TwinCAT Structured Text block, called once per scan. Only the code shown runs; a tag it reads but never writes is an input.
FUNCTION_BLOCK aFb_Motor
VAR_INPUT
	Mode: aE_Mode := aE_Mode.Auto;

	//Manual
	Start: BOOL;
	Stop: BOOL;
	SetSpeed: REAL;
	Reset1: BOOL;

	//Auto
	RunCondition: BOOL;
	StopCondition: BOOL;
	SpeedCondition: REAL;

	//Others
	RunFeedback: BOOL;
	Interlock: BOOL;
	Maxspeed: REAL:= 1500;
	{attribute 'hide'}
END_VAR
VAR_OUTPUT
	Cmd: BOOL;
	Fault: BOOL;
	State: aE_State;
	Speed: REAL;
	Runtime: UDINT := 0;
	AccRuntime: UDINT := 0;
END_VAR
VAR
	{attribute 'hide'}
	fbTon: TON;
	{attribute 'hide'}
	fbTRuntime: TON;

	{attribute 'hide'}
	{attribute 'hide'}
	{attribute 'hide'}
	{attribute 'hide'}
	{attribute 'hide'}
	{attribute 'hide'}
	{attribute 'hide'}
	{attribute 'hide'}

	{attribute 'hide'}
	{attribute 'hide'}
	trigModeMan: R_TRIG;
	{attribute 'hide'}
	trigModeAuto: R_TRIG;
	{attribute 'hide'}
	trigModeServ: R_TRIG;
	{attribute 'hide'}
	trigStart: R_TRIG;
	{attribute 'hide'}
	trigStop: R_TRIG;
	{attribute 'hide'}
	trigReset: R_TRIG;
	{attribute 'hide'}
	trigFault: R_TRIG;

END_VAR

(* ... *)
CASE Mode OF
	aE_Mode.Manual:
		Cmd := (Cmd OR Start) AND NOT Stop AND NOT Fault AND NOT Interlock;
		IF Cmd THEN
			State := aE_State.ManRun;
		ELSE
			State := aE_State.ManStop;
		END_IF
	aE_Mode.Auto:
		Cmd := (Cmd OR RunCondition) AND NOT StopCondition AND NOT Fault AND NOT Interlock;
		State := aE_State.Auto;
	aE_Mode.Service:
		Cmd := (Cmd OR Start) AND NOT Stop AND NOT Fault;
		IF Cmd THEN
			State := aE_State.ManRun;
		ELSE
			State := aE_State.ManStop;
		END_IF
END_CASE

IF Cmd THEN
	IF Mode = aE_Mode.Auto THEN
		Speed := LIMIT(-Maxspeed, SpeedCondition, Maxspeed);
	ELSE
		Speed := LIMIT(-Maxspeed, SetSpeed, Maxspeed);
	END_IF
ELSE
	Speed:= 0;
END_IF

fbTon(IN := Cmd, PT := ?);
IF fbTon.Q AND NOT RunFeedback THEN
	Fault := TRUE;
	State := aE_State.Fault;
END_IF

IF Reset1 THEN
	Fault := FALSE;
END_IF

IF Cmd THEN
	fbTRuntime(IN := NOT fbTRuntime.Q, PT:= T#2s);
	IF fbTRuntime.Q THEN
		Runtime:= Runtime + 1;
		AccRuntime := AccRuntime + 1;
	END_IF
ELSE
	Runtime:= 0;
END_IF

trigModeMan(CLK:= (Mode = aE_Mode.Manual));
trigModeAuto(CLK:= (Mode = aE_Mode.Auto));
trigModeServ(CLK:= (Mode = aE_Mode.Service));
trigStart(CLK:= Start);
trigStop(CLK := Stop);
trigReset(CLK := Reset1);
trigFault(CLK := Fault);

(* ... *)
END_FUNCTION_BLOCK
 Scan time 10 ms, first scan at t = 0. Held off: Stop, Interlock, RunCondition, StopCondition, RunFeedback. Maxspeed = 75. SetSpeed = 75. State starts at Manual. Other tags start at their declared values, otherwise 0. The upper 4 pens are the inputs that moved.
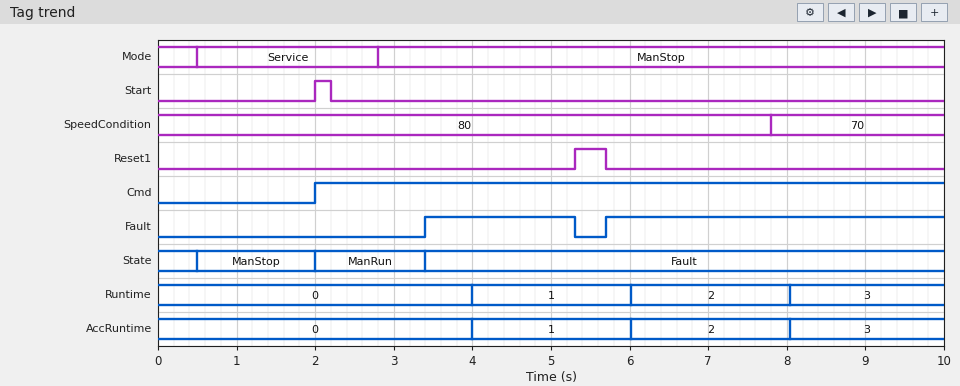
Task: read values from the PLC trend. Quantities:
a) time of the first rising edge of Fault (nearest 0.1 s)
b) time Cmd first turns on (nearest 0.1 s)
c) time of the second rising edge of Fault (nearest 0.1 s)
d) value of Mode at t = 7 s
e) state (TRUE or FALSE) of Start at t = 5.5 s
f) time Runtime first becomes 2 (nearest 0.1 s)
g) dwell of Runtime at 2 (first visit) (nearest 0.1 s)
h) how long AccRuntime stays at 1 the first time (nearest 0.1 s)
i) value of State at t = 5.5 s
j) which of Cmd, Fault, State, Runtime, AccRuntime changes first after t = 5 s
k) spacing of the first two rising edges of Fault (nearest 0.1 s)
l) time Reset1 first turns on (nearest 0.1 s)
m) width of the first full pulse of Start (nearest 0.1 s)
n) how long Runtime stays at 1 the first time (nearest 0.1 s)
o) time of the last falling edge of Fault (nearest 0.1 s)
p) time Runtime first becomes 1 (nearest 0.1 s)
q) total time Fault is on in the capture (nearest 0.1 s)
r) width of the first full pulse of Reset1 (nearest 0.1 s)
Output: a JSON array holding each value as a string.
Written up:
["3.4 s", "2.0 s", "5.7 s", "ManStop", "FALSE", "6.0 s", "2.0 s", "2.0 s", "Fault", "Fault", "2.3 s", "5.3 s", "0.2 s", "2.0 s", "5.3 s", "4.0 s", "6.2 s", "0.4 s"]
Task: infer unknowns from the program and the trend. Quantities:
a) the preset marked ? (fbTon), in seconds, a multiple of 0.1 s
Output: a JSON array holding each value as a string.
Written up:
["1.4 s"]
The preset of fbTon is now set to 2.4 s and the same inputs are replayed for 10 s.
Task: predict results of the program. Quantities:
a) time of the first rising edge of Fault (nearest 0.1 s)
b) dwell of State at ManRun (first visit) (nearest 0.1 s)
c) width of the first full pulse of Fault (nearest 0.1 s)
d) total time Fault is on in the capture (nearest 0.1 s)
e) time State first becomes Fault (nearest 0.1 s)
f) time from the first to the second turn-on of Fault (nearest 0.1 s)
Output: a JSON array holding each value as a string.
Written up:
["4.4 s", "2.4 s", "0.9 s", "5.2 s", "4.4 s", "1.3 s"]
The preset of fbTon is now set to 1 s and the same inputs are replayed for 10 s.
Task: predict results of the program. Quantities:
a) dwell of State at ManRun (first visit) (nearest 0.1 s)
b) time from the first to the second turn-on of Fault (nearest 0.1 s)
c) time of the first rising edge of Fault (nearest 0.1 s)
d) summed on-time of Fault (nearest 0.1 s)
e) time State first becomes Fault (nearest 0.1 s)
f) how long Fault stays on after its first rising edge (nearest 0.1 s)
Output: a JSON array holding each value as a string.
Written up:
["1.0 s", "2.7 s", "3.0 s", "6.6 s", "3.0 s", "2.3 s"]
